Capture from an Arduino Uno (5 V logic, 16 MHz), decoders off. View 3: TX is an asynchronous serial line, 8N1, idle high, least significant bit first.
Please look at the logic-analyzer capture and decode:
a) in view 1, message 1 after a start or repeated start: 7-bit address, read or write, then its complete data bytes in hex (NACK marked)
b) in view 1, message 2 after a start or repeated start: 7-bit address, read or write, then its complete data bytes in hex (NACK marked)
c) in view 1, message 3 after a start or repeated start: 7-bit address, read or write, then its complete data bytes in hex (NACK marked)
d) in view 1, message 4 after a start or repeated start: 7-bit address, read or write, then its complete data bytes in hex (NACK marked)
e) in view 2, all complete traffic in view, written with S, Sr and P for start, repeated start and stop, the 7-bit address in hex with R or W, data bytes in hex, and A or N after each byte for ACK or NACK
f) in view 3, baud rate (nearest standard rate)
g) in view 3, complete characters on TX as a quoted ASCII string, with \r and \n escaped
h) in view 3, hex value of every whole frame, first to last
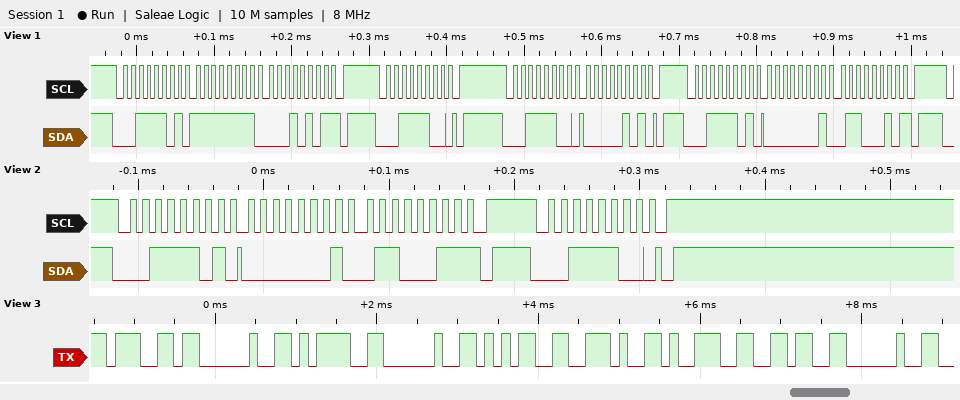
0x1E read: FF 15 NACK
0x1E write
0x1E write: 05
0x1E read: 01 62 NACK
S 1ER A 01 A 63 N P S 1EW A P
9600 baud
"g = 5.96 "
67 20 3D 20 35 2E 39 36 20
